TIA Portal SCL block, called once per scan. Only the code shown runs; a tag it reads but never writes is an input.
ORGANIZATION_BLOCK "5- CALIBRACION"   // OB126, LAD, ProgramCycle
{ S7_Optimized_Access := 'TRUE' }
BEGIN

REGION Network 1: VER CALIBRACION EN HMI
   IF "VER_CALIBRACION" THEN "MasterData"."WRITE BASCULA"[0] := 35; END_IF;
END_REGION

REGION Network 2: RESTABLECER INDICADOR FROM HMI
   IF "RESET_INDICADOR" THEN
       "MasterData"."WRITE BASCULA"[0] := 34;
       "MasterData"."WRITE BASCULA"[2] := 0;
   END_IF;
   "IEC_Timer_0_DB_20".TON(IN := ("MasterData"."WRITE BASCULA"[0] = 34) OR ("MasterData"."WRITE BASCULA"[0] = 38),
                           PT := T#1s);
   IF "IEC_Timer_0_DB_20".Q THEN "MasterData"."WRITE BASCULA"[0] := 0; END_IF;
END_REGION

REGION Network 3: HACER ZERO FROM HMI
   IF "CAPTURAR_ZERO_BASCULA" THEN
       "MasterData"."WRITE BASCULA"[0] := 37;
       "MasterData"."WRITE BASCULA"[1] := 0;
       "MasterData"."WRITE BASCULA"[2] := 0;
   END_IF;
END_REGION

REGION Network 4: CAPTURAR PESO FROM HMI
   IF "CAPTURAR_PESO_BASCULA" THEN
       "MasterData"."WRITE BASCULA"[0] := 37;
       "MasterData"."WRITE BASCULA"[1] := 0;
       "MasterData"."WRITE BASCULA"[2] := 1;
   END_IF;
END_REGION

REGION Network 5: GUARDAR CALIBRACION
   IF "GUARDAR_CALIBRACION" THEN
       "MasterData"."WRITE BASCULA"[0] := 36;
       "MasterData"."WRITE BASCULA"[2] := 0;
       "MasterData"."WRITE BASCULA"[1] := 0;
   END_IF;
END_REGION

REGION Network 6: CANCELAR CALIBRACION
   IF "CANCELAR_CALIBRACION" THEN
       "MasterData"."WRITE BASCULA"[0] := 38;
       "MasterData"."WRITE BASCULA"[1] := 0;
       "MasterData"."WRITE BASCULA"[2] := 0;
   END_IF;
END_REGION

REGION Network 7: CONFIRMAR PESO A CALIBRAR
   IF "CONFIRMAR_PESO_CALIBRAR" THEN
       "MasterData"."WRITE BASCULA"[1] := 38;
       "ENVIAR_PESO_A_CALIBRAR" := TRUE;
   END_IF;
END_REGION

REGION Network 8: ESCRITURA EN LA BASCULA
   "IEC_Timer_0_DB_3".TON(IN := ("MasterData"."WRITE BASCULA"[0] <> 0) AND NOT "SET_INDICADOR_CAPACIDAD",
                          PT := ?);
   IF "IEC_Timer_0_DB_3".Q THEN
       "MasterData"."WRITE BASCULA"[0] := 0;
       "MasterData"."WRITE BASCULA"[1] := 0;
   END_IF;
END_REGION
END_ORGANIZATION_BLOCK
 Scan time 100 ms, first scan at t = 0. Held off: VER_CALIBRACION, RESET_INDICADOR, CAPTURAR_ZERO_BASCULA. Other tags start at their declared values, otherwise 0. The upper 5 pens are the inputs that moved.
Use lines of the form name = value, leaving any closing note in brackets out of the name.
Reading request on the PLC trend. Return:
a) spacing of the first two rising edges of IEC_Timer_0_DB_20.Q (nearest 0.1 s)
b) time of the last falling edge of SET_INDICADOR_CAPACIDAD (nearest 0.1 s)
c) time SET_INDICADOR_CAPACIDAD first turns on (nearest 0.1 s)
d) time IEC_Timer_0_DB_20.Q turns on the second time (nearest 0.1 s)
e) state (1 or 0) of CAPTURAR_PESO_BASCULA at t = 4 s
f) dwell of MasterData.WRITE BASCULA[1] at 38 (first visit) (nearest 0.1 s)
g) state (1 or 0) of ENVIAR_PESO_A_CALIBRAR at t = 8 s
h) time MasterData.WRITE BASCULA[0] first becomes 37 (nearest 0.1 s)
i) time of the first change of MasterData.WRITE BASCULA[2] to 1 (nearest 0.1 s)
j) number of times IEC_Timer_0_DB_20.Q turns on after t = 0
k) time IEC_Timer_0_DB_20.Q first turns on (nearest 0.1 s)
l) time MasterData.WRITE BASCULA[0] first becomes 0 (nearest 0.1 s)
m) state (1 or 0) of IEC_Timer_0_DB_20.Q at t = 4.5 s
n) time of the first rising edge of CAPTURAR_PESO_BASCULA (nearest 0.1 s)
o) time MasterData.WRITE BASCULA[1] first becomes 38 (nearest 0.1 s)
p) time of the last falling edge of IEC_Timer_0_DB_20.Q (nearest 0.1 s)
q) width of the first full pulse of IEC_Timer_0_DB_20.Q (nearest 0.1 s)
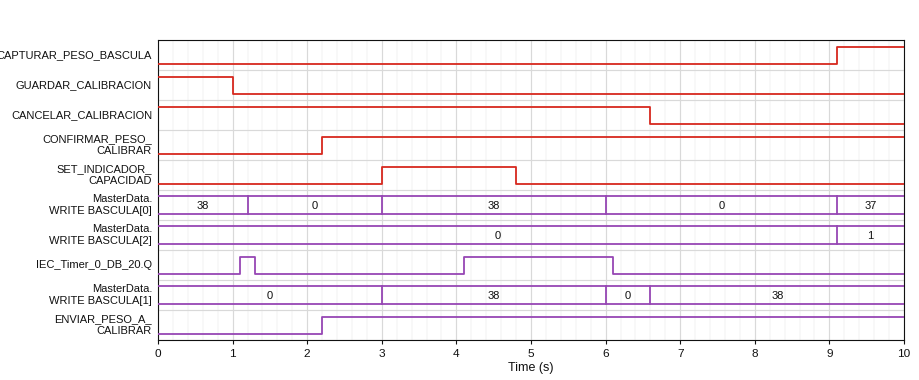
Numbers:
spacing of the first two rising edges of IEC_Timer_0_DB_20.Q = 3.0 s
time of the last falling edge of SET_INDICADOR_CAPACIDAD = 4.8 s
time SET_INDICADOR_CAPACIDAD first turns on = 3.0 s
time IEC_Timer_0_DB_20.Q turns on the second time = 4.1 s
state (1 or 0) of CAPTURAR_PESO_BASCULA at t = 4 s = 0
dwell of MasterData.WRITE BASCULA[1] at 38 (first visit) = 3.0 s
state (1 or 0) of ENVIAR_PESO_A_CALIBRAR at t = 8 s = 1
time MasterData.WRITE BASCULA[0] first becomes 37 = 9.1 s
time of the first change of MasterData.WRITE BASCULA[2] to 1 = 9.1 s
number of times IEC_Timer_0_DB_20.Q turns on after t = 0 = 2
time IEC_Timer_0_DB_20.Q first turns on = 1.1 s
time MasterData.WRITE BASCULA[0] first becomes 0 = 1.2 s
state (1 or 0) of IEC_Timer_0_DB_20.Q at t = 4.5 s = 1
time of the first rising edge of CAPTURAR_PESO_BASCULA = 9.1 s
time MasterData.WRITE BASCULA[1] first becomes 38 = 3.0 s
time of the last falling edge of IEC_Timer_0_DB_20.Q = 6.1 s
width of the first full pulse of IEC_Timer_0_DB_20.Q = 0.2 s
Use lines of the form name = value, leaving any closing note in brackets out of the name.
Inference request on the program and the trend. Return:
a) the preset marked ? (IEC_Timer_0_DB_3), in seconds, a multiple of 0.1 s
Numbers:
the preset marked ? (IEC_Timer_0_DB_3), in seconds, a multiple of 0.1 s = 1.2 s
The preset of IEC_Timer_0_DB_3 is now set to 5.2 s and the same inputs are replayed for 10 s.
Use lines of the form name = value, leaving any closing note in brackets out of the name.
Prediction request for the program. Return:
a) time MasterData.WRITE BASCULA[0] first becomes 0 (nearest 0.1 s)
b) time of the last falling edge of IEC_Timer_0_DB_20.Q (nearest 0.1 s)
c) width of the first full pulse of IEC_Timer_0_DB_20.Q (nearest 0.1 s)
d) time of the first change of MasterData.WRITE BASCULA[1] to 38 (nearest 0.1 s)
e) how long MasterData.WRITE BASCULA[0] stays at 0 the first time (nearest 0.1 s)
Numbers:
time MasterData.WRITE BASCULA[0] first becomes 0 = 6.6 s
time of the last falling edge of IEC_Timer_0_DB_20.Q = 6.7 s
width of the first full pulse of IEC_Timer_0_DB_20.Q = 5.6 s
time of the first change of MasterData.WRITE BASCULA[1] to 38 = 2.2 s
how long MasterData.WRITE BASCULA[0] stays at 0 the first time = 2.5 s
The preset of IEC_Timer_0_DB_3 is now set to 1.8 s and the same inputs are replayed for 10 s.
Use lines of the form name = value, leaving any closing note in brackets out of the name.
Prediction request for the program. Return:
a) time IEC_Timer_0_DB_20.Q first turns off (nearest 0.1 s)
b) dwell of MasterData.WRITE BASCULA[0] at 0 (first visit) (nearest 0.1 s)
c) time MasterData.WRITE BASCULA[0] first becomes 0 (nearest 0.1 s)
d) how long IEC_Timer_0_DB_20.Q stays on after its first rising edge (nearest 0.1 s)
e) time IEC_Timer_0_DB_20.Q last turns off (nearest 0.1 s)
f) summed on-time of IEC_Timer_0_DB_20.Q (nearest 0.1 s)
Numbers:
time IEC_Timer_0_DB_20.Q first turns off = 1.9 s
dwell of MasterData.WRITE BASCULA[0] at 0 (first visit) = 1.2 s
time MasterData.WRITE BASCULA[0] first becomes 0 = 1.8 s
how long IEC_Timer_0_DB_20.Q stays on after its first rising edge = 0.8 s
time IEC_Timer_0_DB_20.Q last turns off = 6.7 s
summed on-time of IEC_Timer_0_DB_20.Q = 3.4 s
